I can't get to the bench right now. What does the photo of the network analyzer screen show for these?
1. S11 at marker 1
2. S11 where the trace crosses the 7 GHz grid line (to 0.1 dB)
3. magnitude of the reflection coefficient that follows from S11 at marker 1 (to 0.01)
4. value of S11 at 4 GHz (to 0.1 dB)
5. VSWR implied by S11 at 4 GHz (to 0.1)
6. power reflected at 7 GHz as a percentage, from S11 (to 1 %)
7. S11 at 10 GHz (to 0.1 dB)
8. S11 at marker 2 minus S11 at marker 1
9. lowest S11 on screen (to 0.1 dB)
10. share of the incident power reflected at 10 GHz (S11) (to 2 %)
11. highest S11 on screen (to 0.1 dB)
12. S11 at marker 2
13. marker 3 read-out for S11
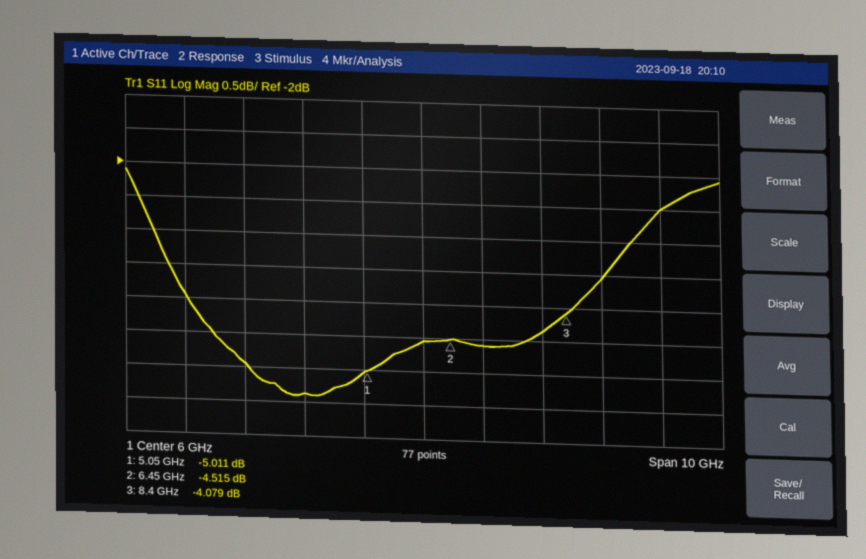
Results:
-5.011 dB
-4.6 dB
0.56
-5.4 dB
3.3
35 %
-2.5 dB
0.496 dB
-5.4 dB
56 %
-2.1 dB
-4.515 dB
-4.079 dB
